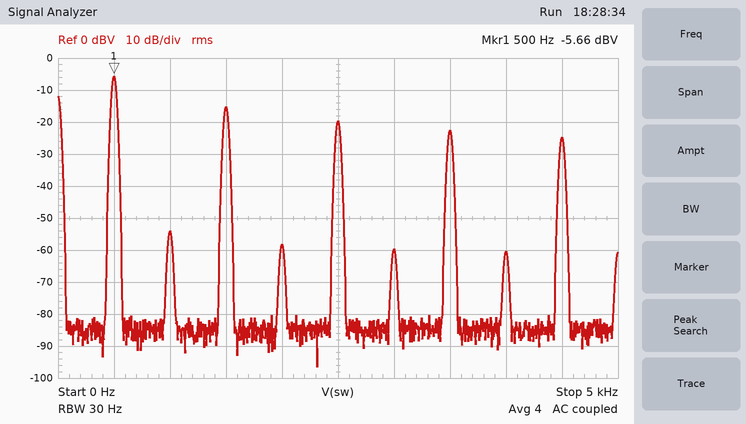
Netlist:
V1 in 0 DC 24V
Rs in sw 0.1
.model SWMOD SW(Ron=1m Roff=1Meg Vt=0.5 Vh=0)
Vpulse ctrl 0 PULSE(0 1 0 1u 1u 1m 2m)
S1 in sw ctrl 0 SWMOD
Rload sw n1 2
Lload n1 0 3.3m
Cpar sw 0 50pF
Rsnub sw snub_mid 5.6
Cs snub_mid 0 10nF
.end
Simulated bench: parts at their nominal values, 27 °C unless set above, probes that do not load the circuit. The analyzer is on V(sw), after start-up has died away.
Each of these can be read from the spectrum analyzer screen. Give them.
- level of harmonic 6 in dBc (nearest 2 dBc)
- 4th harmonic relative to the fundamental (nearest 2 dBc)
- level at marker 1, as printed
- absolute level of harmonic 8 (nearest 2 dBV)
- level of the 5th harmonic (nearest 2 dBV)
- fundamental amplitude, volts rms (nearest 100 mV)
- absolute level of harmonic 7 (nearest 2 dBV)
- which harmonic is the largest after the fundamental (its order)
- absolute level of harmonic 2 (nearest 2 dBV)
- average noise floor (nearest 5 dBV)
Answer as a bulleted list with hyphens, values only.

- -54 dBc
- -52 dBc
- -5.66 dBV
- -60 dBV
- -20 dBV
- 500 mV
- -22 dBV
- 3
- -54 dBV
- -85 dBV
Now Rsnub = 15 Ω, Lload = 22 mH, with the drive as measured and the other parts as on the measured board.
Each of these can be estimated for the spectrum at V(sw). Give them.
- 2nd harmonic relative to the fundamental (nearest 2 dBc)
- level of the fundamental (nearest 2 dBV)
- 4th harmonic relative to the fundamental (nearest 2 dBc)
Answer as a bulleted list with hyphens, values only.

- -56 dBc
- -6 dBV
- -56 dBc
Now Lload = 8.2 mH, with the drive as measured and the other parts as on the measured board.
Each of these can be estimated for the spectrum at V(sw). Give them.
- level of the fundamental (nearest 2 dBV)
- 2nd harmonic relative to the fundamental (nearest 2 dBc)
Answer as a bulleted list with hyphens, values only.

- -6 dBV
- -54 dBc
